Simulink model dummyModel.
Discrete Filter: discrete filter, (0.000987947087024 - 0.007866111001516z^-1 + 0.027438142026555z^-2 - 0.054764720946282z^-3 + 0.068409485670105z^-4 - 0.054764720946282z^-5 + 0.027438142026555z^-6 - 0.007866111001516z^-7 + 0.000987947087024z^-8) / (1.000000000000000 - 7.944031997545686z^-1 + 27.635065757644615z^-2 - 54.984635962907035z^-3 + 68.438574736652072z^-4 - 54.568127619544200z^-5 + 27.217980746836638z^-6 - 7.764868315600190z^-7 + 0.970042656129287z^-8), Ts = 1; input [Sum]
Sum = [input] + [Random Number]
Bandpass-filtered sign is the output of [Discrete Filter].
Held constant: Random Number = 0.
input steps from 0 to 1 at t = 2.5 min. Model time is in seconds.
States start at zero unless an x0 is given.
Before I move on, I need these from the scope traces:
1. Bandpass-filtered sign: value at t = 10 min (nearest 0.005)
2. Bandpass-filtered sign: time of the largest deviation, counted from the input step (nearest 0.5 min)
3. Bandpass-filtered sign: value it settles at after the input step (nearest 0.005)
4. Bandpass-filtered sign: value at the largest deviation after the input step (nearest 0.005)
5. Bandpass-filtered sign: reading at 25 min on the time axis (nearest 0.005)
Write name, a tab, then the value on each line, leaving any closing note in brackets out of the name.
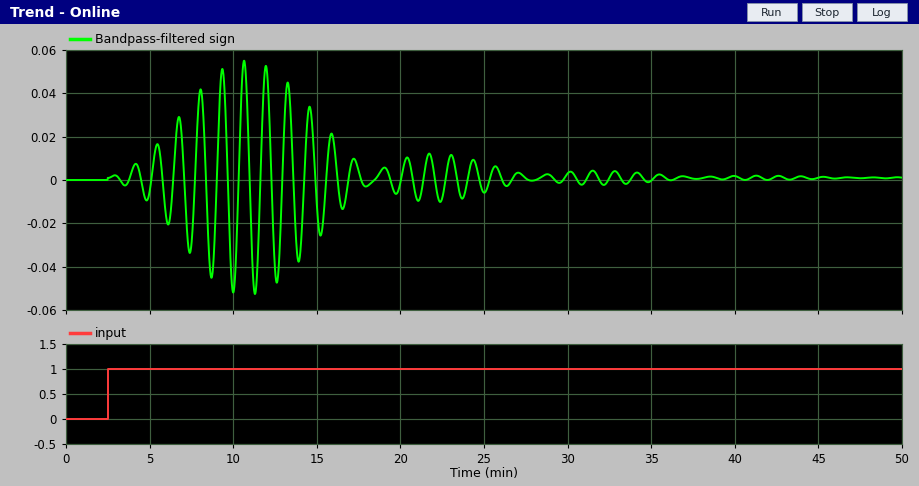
Bandpass-filtered sign: value at t = 10 min	-0.050
Bandpass-filtered sign: time of the largest deviation, counted from the input step	8.0 min
Bandpass-filtered sign: value it settles at after the input step	0.000
Bandpass-filtered sign: value at the largest deviation after the input step	0.055
Bandpass-filtered sign: reading at 25 min on the time axis	-0.005
